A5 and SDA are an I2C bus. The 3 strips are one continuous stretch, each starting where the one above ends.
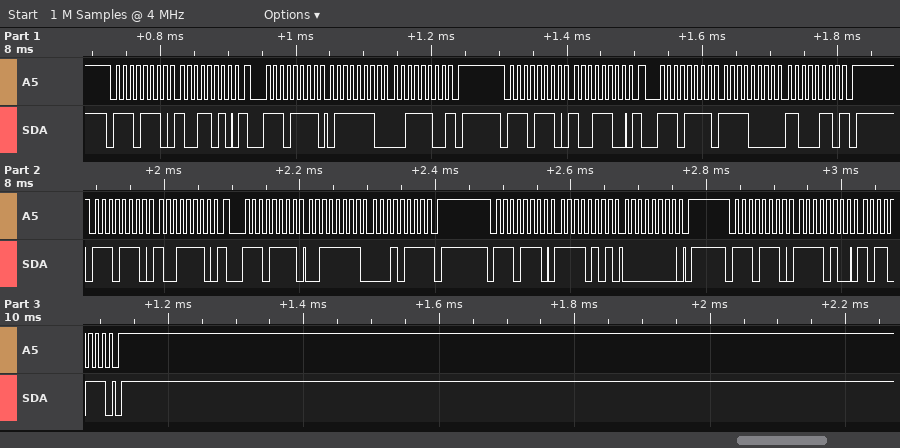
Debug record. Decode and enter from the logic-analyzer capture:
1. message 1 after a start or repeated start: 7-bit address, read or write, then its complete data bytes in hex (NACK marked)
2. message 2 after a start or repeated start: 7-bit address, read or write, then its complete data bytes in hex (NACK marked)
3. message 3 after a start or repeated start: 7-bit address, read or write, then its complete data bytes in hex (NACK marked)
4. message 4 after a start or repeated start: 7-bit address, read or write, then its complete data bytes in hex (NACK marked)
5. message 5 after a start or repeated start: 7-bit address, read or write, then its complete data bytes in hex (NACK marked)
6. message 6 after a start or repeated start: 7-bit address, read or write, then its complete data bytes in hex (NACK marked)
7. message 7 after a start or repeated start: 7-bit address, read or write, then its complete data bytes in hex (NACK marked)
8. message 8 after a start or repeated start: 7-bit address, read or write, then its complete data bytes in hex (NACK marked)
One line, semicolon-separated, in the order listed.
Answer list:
0x77 write: 9A; 0x77 read: 7E 3C NACK; 0x77 write: 9C; 0x77 read: F0 C6 NACK; 0x77 write: 9E; 0x77 read: 3F 17 NACK; 0x77 write: F5 00; 0x77 write: F4 B7
